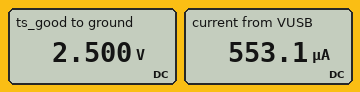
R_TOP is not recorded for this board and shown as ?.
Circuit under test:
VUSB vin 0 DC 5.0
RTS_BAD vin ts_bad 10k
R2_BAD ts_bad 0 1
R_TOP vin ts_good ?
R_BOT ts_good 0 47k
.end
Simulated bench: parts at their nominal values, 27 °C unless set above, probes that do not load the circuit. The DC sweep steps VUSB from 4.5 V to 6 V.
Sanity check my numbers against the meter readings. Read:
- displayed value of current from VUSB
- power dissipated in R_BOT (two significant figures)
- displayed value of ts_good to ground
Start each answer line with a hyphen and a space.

- 553.1 µA
- 130 µW
- 2.500 V
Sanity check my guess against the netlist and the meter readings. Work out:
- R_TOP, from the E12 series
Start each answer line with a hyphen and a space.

- 47 kΩ
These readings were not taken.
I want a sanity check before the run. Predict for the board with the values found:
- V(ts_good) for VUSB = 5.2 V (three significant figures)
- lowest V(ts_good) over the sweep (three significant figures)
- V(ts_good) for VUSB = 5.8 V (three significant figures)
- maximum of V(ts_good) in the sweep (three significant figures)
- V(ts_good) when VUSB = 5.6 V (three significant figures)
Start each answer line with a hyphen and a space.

- 2.60 V
- 2.25 V
- 2.90 V
- 3.00 V
- 2.80 V
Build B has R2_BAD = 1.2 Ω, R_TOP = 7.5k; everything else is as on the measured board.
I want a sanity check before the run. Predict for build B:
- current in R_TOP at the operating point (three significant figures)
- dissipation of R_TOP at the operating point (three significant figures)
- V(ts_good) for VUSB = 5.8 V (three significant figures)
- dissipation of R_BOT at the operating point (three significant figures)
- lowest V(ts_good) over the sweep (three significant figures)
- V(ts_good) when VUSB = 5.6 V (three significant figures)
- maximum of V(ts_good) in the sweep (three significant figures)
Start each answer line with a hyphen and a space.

- 91.7 µA
- 63.1 µW
- 5.00 V
- 396 µW
- 3.88 V
- 4.83 V
- 5.17 V
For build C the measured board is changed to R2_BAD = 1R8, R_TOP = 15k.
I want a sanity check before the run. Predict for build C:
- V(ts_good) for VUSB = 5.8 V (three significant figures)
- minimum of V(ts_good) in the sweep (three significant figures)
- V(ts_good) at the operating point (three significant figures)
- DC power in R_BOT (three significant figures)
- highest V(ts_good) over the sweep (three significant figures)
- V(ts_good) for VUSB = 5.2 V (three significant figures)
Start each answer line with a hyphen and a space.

- 4.40 V
- 3.41 V
- 3.79 V
- 306 µW
- 4.55 V
- 3.94 V
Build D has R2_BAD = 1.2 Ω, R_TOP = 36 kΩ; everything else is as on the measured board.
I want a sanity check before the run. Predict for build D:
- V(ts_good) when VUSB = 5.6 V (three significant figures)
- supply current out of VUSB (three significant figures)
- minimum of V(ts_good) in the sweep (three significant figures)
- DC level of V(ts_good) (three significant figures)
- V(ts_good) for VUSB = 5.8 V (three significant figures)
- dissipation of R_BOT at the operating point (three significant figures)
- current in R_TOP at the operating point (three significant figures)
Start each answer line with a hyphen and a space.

- 3.17 V
- 560 µA
- 2.55 V
- 2.83 V
- 3.28 V
- 171 µW
- 60.2 µA
